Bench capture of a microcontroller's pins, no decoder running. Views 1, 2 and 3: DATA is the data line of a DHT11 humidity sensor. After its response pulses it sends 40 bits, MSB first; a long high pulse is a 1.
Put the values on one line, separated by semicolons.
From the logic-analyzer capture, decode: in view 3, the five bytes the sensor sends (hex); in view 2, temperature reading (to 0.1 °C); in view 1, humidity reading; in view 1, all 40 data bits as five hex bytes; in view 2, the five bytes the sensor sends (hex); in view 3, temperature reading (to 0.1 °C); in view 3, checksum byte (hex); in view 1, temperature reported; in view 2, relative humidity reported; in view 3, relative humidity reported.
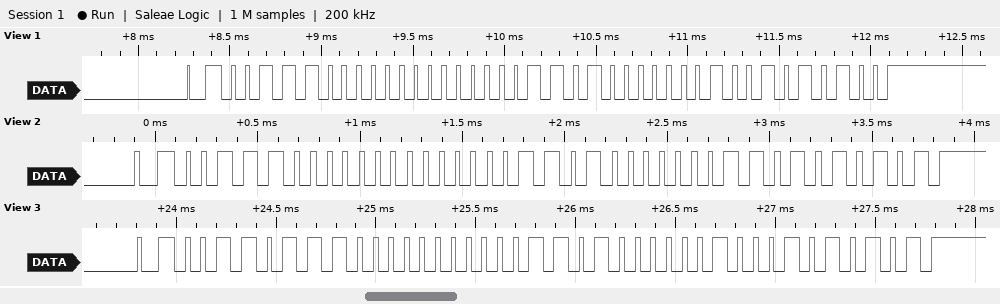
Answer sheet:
37 00 1A 04 55; 26.3 °C; 56 %; 38 00 1A 02 54; 38 00 1A 03 55; 26.4 °C; 0x55; 26.2 °C; 56 %; 55 %
